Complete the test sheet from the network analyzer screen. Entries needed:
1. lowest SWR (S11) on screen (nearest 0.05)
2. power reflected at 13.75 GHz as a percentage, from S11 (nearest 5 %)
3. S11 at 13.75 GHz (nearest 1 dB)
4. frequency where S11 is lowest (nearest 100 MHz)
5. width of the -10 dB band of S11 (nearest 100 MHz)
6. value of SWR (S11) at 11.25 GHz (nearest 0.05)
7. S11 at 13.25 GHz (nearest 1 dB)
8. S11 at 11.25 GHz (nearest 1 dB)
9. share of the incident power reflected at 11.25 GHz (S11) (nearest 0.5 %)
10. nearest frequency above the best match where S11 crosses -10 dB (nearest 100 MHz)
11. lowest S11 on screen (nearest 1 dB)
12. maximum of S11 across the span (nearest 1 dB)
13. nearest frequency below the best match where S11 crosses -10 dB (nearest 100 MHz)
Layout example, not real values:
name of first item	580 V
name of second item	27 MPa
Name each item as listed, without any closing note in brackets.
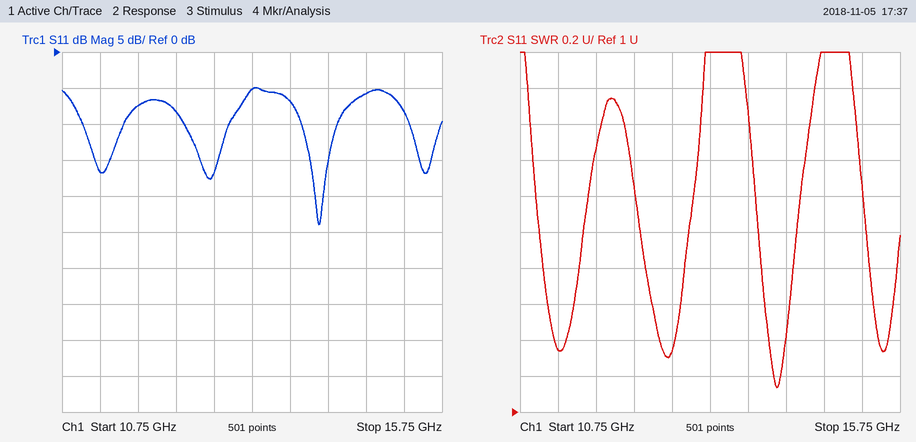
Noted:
lowest SWR (S11) on screen	1.15
power reflected at 13.75 GHz as a percentage, from S11	20 %
S11 at 13.75 GHz	-7 dB
frequency where S11 is lowest	14.1 GHz
width of the -10 dB band of S11	500 MHz
value of SWR (S11) at 11.25 GHz	1.35
S11 at 13.25 GHz	-5 dB
S11 at 11.25 GHz	-17 dB
share of the incident power reflected at 11.25 GHz (S11)	2.0 %
nearest frequency above the best match where S11 crosses -10 dB	14.4 GHz
lowest S11 on screen	-24 dB
maximum of S11 across the span	-5 dB
nearest frequency below the best match where S11 crosses -10 dB	13.9 GHz
